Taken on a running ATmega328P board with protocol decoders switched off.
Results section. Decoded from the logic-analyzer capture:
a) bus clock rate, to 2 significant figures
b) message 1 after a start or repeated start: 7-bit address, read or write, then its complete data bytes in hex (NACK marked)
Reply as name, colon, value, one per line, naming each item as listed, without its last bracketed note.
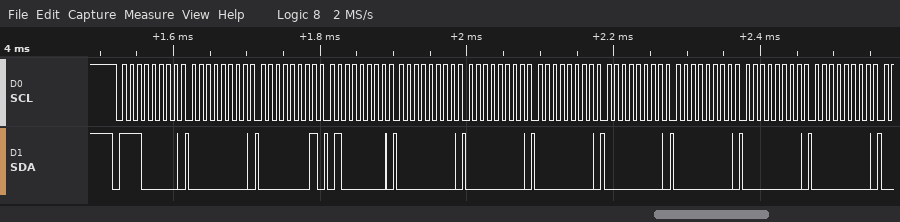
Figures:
bus clock rate, to 2 significant figures: 100 kHz
message 1 after a start or repeated start: 7-bit address, read or write, then its complete data bytes in hex: 0x70 write: 00 01 40 00 00 00 00 00 00 00
